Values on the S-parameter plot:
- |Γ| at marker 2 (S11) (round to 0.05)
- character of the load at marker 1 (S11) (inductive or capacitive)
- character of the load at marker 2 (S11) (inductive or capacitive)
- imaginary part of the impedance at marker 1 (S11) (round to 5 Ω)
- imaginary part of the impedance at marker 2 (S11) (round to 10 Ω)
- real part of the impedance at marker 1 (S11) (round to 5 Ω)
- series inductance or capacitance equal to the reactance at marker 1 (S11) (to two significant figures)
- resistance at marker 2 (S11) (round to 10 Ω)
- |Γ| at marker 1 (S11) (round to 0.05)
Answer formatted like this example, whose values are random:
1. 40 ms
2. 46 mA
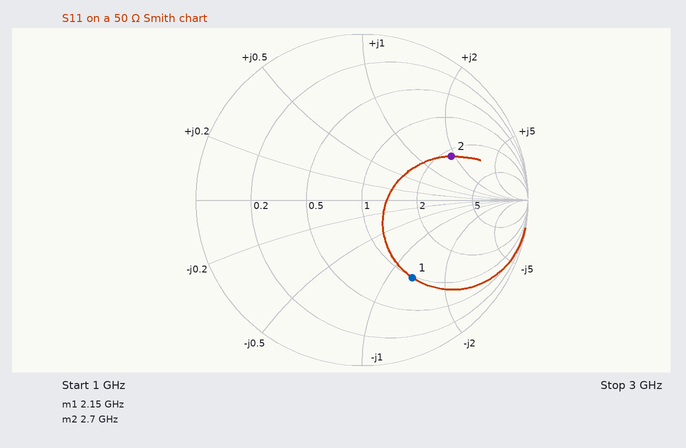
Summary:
1. 0.60
2. capacitive
3. inductive
4. -65 Ω
5. +90 Ω
6. 50 Ω
7. 1.1 pF
8. 110 Ω
9. 0.55
